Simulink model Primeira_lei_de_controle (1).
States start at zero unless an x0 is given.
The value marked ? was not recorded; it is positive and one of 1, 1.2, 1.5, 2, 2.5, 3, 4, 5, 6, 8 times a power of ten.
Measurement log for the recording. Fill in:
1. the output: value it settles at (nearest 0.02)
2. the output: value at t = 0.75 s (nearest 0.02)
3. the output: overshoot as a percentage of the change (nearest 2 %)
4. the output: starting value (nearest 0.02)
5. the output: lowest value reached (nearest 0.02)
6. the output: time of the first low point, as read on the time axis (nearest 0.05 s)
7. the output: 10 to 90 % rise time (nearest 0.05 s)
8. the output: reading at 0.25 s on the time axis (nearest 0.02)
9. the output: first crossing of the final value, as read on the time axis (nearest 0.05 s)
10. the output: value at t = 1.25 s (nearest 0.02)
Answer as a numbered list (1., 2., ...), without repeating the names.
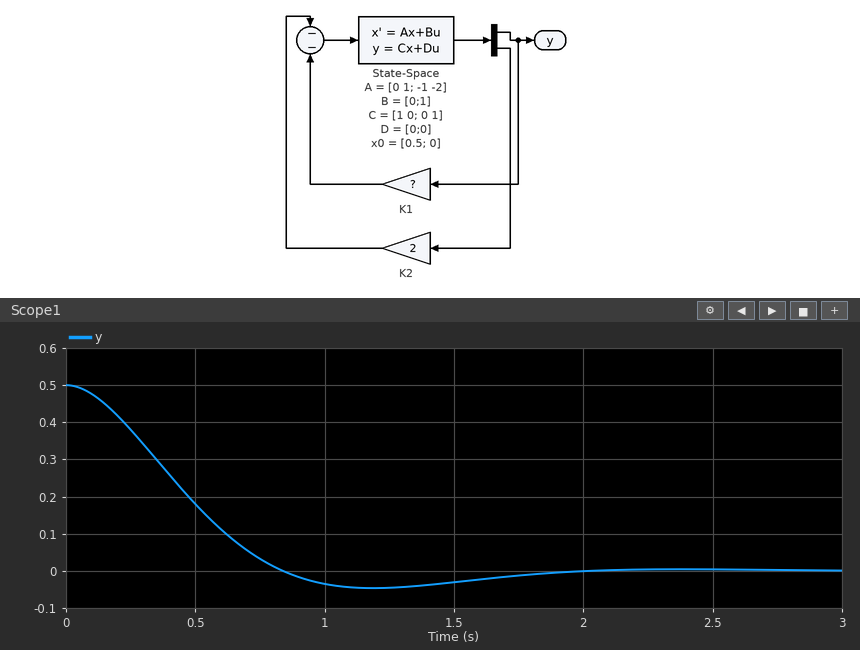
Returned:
1. 0.00
2. 0.04
3. 10 %
4. 0.50
5. -0.04
6. 1.20 s
7. 0.55 s
8. 0.38
9. 0.85 s
10. -0.04
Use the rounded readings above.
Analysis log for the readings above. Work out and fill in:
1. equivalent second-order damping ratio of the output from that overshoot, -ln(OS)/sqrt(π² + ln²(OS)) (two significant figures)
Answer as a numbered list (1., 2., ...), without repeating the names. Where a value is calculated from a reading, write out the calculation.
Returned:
1. ln(0.1) = -2.303; 2.303 / sqrt(9.870 + 5.302) = 0.59
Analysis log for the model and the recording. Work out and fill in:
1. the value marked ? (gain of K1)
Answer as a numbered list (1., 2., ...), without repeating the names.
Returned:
1. 10
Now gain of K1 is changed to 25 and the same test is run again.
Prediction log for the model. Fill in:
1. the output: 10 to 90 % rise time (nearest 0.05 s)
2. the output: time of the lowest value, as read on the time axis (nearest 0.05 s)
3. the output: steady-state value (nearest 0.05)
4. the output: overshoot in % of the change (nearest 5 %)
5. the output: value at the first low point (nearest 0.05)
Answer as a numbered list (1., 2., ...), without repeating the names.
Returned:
1. 0.30 s
2. 0.65 s
3. 0.00
4. 25 %
5. -0.15
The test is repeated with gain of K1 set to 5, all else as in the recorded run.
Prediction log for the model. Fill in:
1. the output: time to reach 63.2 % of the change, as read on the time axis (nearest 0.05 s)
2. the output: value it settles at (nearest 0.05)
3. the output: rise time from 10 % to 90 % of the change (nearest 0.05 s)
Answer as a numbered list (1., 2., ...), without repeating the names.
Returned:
1. 0.75 s
2. 0.00
3. 1.05 s
